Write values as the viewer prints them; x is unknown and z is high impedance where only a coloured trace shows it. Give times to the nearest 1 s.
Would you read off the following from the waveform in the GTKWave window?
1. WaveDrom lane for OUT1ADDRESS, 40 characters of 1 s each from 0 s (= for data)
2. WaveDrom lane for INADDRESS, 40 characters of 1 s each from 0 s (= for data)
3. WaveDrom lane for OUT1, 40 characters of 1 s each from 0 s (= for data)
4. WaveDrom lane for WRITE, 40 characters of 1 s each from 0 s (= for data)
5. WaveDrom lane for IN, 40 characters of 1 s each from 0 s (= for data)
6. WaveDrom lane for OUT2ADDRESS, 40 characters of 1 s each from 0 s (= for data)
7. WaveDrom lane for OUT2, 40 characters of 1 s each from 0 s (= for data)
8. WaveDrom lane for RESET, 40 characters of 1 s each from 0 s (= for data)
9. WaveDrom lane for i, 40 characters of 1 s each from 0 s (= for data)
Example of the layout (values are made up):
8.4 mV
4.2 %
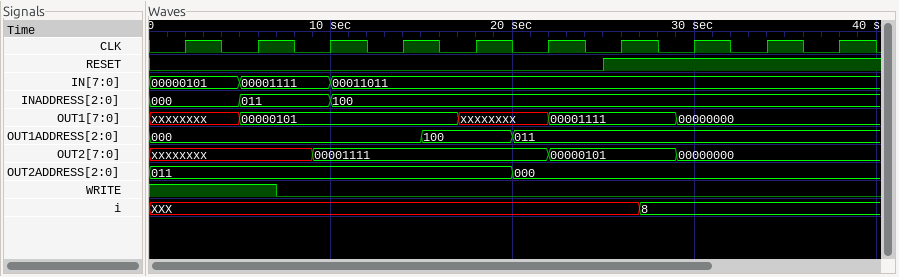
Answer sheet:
{name: 'OUT1ADDRESS', wave: '=..............=....=...................', data: '000 100 011'}
{name: 'INADDRESS', wave: '=....=....=.............................', data: '000 011 100'}
{name: 'OUT1', wave: 'x....=...........x....=......=..........', data: '00000101 00001111 00000000'}
{name: 'WRITE', wave: '1......0................................'}
{name: 'IN', wave: '=....=....=.............................', data: '00000101 00001111 00011011'}
{name: 'OUT2ADDRESS', wave: '=...................=...................', data: '011 000'}
{name: 'OUT2', wave: 'x........=............=......=..........', data: '00001111 00000101 00000000'}
{name: 'RESET', wave: '0........................1..............'}
{name: 'i', wave: 'x..........................=............', data: '8'}
